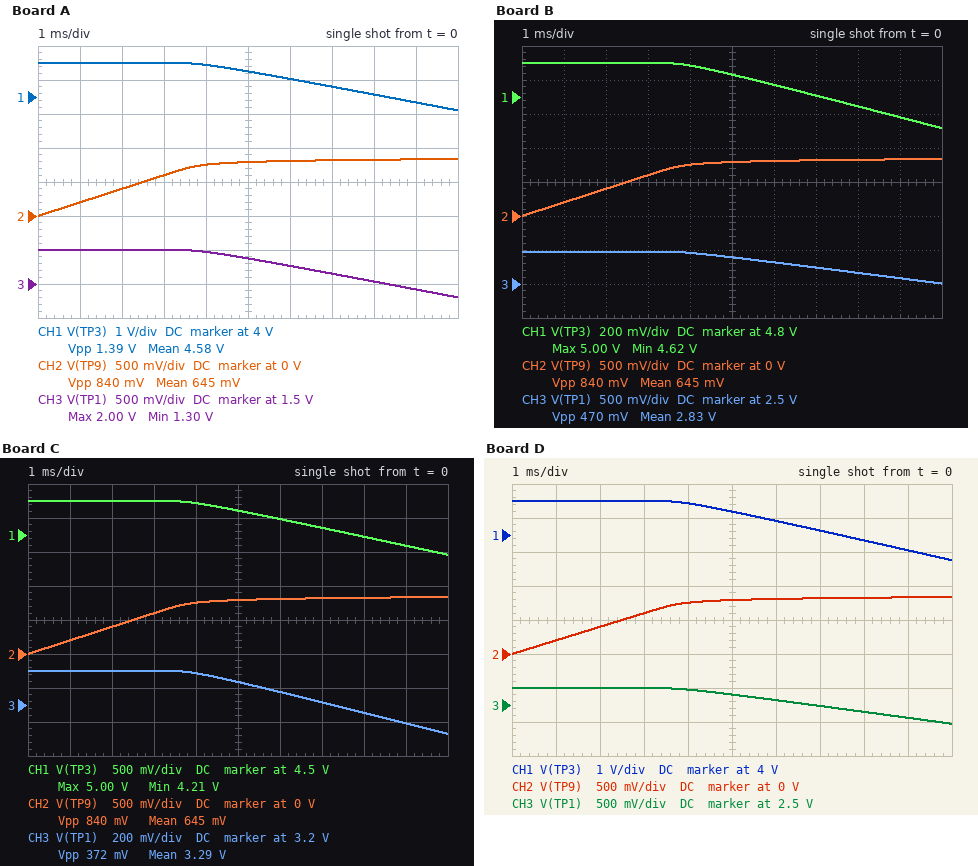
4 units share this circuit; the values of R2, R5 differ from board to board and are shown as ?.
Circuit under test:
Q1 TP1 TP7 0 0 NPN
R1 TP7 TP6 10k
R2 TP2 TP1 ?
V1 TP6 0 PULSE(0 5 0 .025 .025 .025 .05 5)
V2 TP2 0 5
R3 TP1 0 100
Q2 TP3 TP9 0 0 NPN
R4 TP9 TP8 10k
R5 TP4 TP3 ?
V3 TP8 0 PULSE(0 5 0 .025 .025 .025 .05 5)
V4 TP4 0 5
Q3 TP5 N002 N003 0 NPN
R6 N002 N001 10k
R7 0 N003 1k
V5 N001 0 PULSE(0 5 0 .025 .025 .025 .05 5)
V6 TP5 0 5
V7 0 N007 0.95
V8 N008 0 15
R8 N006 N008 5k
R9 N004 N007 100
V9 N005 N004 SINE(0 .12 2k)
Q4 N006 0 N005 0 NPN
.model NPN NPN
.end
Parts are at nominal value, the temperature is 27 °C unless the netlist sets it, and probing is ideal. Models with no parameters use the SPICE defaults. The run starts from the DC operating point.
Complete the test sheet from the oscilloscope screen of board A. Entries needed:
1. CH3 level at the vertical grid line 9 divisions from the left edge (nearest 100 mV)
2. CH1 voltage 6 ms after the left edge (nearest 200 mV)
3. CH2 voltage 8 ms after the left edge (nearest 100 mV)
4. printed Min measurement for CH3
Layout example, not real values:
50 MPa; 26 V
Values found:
1.4 V; 4.6 V; 800 mV; 1.30 V
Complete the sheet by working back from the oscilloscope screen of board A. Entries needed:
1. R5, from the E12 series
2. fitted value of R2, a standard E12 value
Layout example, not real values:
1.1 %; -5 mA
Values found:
120 Ω; 150 Ω
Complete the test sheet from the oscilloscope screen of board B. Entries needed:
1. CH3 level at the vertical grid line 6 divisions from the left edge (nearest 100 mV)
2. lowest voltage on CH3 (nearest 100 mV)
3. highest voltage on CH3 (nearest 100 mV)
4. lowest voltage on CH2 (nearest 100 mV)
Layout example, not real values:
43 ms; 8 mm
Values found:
2.8 V; 2.5 V; 3.0 V; 0 V
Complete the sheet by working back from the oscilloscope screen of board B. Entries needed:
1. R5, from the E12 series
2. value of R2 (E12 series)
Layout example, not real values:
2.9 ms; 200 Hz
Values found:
33 Ω; 68 Ω
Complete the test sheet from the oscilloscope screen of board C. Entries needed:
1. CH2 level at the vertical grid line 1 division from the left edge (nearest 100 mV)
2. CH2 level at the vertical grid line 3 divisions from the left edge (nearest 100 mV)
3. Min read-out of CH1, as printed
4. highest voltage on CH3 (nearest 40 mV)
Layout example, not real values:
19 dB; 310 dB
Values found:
200 mV; 600 mV; 4.21 V; 3.40 V
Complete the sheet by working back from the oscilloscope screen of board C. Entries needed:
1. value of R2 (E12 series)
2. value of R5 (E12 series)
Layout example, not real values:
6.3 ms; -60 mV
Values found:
47 Ω; 68 Ω
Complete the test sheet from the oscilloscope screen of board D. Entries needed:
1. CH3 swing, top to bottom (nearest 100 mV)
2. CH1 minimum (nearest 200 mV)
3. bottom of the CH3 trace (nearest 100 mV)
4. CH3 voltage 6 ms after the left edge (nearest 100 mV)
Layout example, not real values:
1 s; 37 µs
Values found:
500 mV; 3.2 V; 2.2 V; 2.6 V
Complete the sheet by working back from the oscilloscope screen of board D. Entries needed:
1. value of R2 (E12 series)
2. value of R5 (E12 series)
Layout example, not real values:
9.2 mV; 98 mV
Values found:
82 Ω; 150 Ω
